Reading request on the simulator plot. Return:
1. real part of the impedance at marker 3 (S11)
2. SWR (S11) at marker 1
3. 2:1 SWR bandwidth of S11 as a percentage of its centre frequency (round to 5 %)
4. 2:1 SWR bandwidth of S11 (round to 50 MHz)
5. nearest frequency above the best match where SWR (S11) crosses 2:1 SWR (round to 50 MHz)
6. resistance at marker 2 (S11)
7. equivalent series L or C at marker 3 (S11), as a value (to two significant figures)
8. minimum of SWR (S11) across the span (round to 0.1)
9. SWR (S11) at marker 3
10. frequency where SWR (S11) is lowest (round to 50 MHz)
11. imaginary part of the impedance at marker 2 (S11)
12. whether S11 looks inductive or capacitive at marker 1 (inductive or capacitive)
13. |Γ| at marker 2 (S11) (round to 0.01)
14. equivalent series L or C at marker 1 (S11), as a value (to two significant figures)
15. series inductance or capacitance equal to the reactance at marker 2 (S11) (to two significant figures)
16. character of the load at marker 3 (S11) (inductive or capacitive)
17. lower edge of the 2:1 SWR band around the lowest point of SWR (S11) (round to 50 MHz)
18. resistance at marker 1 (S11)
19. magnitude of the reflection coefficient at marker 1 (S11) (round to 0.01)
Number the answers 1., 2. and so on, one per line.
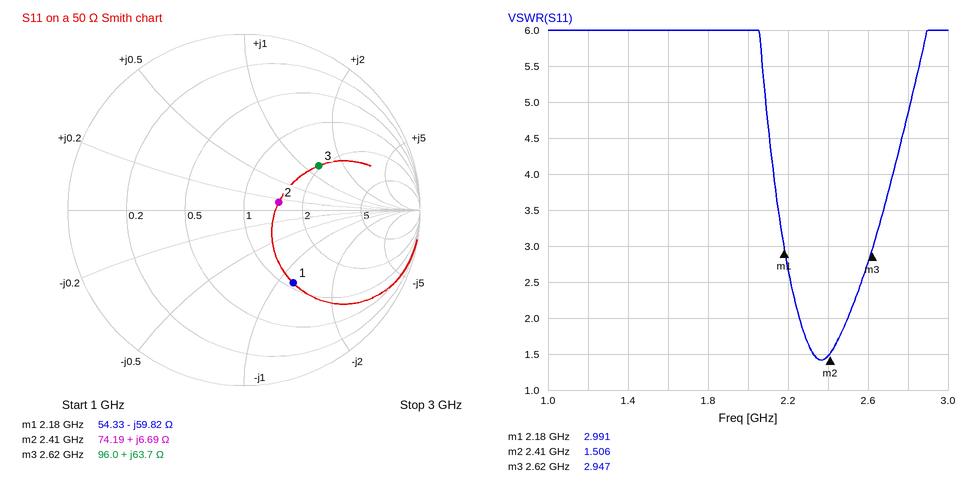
1. 96.0 Ω
2. 2.991
3. 10 %
4. 250 MHz
5. 2.50 GHz
6. 74.19 Ω
7. 3.9 nH
8. 1.4
9. 2.947
10. 2.35 GHz
11. +6.69 Ω
12. capacitive
13. 0.20
14. 1.2 pF
15. 440 pH
16. inductive
17. 2.25 GHz
18. 54.33 Ω
19. 0.50
